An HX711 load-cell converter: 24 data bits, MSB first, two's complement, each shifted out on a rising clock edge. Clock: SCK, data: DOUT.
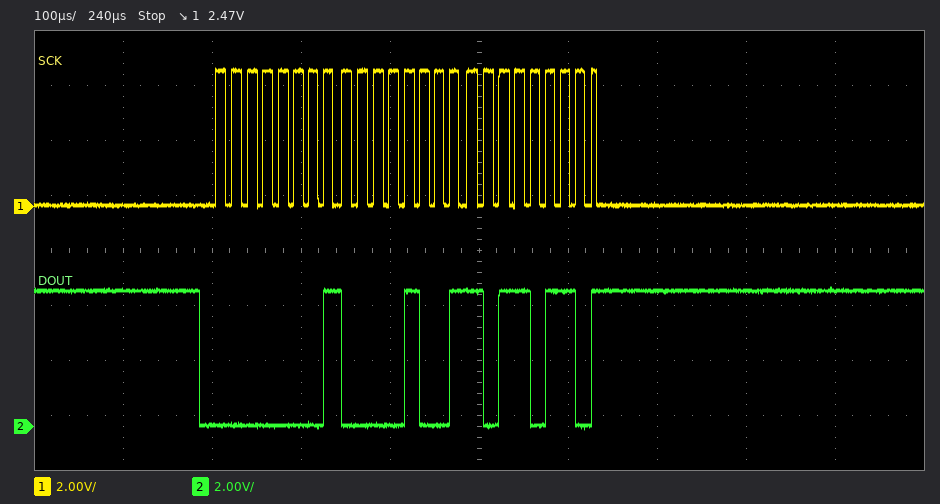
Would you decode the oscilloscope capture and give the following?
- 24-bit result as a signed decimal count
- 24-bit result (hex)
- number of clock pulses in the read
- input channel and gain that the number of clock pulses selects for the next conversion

68022
0x0109B6
25
channel A, gain 128
